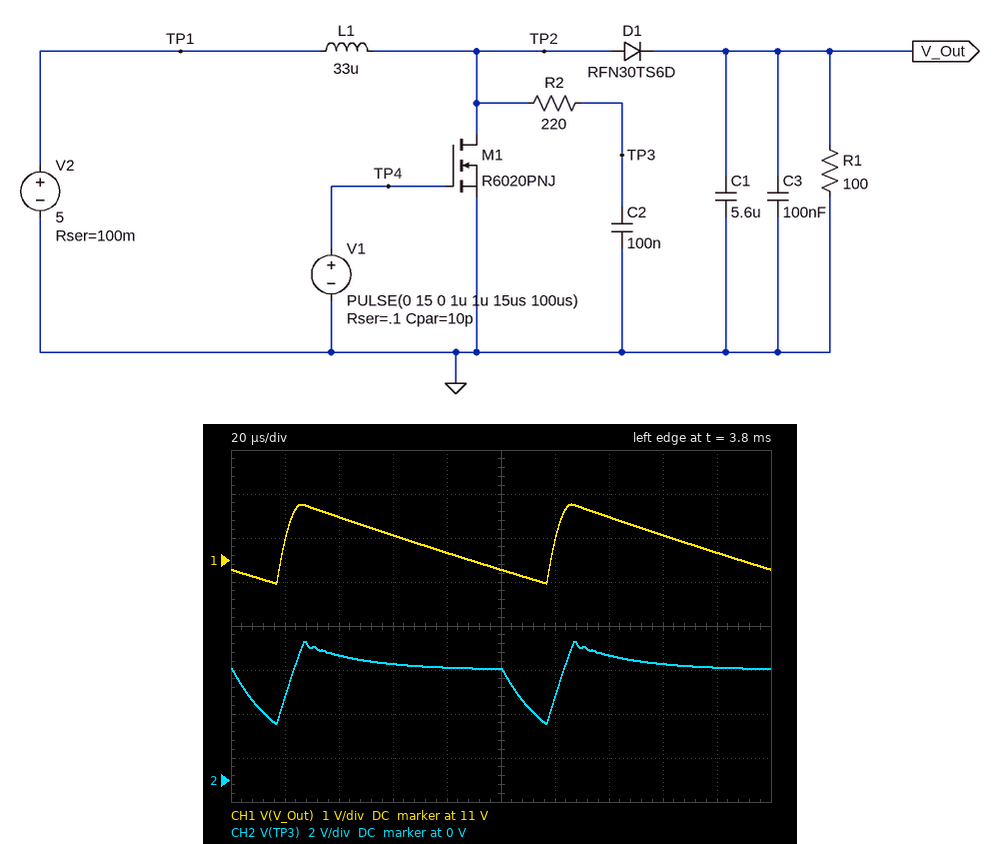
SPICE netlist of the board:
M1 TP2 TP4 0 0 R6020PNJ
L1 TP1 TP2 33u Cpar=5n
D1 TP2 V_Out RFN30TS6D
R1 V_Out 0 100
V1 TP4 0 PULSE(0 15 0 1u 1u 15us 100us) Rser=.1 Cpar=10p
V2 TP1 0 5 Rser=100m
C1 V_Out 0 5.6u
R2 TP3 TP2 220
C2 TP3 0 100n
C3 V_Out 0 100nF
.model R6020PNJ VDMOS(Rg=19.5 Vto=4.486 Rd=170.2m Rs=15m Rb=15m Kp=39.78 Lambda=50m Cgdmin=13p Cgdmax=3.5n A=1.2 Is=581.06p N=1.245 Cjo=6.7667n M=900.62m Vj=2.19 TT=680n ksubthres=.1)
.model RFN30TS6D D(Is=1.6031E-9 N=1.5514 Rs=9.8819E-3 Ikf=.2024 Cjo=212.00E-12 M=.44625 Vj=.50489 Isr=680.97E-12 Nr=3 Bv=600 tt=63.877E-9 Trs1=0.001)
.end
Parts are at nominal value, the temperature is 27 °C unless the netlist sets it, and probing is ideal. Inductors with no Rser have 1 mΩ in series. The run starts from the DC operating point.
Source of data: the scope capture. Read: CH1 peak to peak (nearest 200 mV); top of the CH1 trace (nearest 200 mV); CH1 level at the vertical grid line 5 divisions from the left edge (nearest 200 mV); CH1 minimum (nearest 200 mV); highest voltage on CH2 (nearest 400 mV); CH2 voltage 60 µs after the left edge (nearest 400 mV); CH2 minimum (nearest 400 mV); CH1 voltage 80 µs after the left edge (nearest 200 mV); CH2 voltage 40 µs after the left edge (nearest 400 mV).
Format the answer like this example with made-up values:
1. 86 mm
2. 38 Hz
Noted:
1. 1.8 V
2. 12.2 V
3. 10.8 V
4. 10.4 V
5. 6.4 V
6. 5.2 V
7. 2.4 V
8. 11.2 V
9. 5.6 V
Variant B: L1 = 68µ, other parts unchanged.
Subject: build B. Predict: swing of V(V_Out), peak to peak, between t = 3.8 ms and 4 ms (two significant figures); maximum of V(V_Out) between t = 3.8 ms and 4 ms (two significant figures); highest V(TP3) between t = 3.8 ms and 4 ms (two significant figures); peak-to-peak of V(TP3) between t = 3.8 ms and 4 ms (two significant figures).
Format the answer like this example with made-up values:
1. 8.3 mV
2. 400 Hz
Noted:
1. 1.3 V
2. 9.6 V
3. 6.4 V
4. 3.9 V
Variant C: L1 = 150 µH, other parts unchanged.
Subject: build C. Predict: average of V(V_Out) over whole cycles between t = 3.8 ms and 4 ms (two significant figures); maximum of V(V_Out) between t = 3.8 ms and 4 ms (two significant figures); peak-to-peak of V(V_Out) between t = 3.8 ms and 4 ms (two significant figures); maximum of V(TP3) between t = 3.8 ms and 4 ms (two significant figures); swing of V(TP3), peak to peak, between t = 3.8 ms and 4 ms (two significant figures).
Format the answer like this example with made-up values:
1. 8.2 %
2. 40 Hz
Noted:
1. 7.0 V
2. 7.5 V
3. 930 mV
4. 6.4 V
5. 4.0 V
